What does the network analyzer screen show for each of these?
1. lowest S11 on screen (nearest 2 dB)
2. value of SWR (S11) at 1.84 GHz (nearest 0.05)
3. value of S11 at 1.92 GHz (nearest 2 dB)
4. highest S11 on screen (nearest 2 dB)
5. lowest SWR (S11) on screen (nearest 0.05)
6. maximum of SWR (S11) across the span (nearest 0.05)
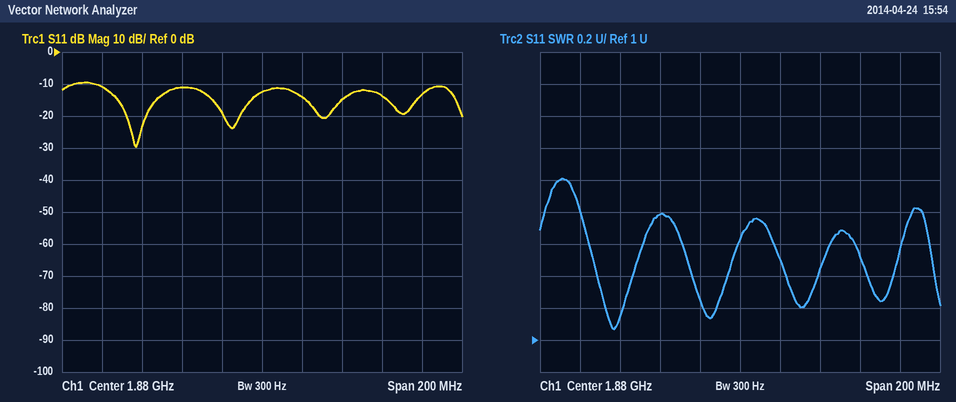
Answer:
-30 dB
1.80
-14 dB
-10 dB
1.05
2.00
